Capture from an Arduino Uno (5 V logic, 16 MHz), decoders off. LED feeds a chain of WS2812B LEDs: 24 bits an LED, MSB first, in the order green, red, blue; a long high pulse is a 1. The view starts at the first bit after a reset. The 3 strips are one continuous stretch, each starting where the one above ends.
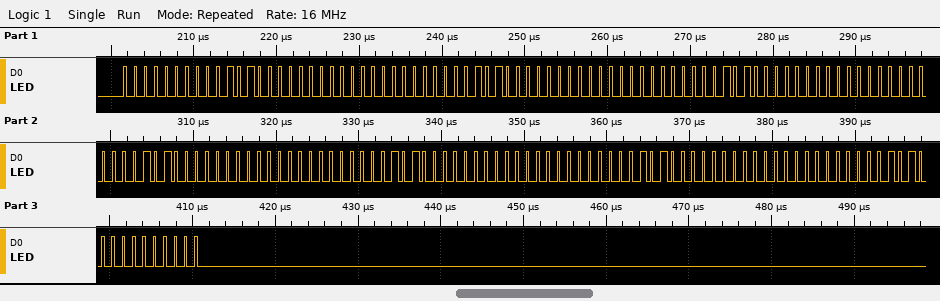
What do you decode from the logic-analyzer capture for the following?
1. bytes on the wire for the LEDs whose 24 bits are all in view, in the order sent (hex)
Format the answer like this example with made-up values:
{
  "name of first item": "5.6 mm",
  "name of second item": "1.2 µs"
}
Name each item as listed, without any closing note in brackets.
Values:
{
  "bytes on the wire for the LEDs whose 24 bits are all in view, in the order sent": "00 28 00 00 28 00 00 28 00 00 28 00 00 28 00 00 28 00 00 28 00"
}
